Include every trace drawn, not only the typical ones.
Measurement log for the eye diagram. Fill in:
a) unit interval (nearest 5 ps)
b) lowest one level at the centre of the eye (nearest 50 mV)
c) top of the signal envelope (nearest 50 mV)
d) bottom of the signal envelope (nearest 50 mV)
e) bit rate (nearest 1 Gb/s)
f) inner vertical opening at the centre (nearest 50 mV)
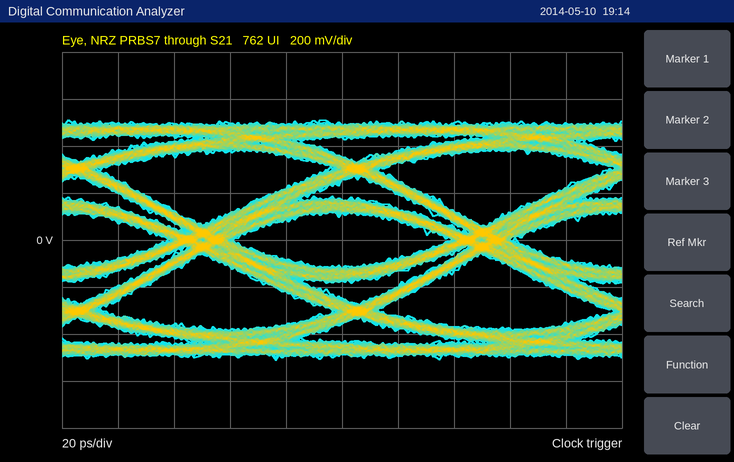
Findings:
100 ps
100 mV
500 mV
-500 mV
10 Gb/s
250 mV
